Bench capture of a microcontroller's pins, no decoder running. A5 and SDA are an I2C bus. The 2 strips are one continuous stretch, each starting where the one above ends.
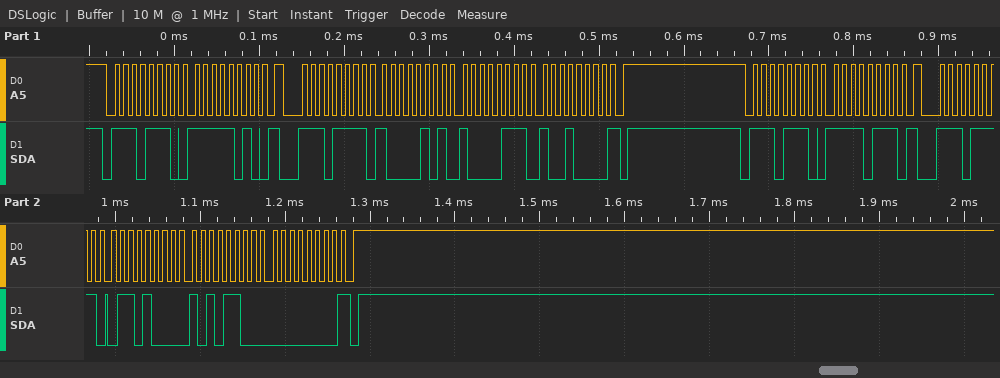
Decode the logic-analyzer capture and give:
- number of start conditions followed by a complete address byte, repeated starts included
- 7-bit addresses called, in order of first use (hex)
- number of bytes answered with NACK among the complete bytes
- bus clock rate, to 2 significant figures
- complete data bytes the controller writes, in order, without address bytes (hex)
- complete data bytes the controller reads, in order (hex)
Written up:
4
0x77
2
100 kHz
FA F7
85 87 90 68 AC 00
